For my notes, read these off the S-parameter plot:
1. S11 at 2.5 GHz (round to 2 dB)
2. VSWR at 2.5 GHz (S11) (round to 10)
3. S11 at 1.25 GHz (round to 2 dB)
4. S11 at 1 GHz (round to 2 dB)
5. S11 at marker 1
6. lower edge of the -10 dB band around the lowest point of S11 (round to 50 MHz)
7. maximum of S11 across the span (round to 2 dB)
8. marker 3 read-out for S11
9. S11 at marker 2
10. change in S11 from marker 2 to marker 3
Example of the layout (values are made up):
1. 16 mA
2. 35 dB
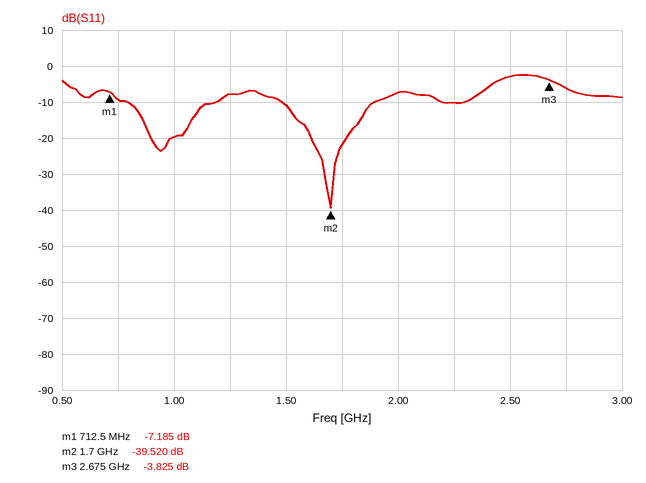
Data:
1. -2 dB
2. 10
3. -8 dB
4. -20 dB
5. -7.185 dB
6. 1.50 GHz
7. -2 dB
8. -3.825 dB
9. -39.520 dB
10. 35.695 dB
